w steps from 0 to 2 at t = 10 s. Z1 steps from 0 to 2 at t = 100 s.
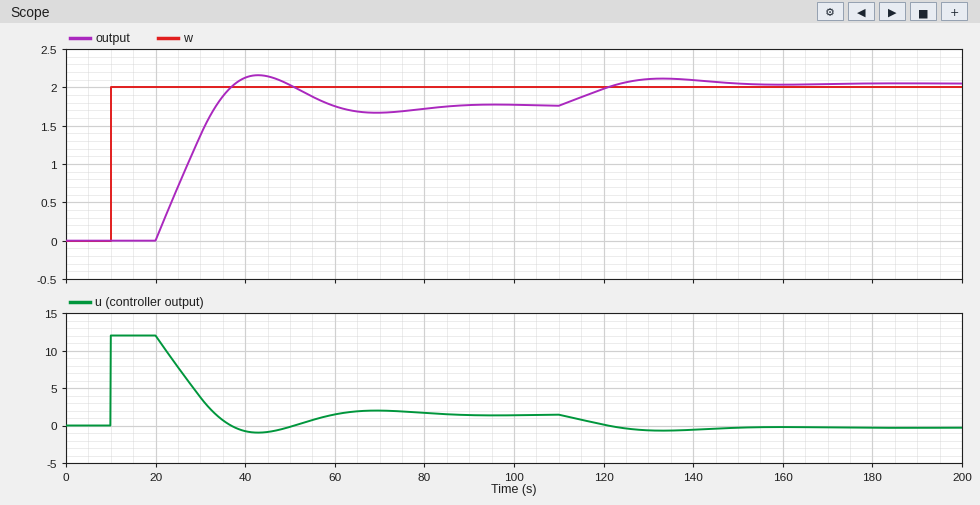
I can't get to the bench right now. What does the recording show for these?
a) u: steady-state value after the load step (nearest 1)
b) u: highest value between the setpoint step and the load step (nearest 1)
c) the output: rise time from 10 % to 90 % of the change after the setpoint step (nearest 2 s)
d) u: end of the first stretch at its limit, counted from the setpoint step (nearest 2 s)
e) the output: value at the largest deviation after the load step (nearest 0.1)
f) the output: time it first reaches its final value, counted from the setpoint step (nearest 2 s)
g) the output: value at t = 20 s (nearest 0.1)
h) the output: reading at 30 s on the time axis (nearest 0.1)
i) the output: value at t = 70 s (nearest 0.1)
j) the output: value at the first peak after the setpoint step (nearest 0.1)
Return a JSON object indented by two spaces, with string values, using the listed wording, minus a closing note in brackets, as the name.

{
  "u: steady-state value after the load step": "0",
  "u: highest value between the setpoint step and the load step": "12",
  "the output: rise time from 10 % to 90 % of the change after the setpoint step": "10 s",
  "u: end of the first stretch at its limit, counted from the setpoint step": "10 s",
  "the output: value at the largest deviation after the load step": "2.1",
  "the output: time it first reaches its final value, counted from the setpoint step": "24 s",
  "the output: value at t = 20 s": "0.0",
  "the output: reading at 30 s on the time axis": "1.4",
  "the output: value at t = 70 s": "1.7",
  "the output: value at the first peak after the setpoint step": "2.2"
}
